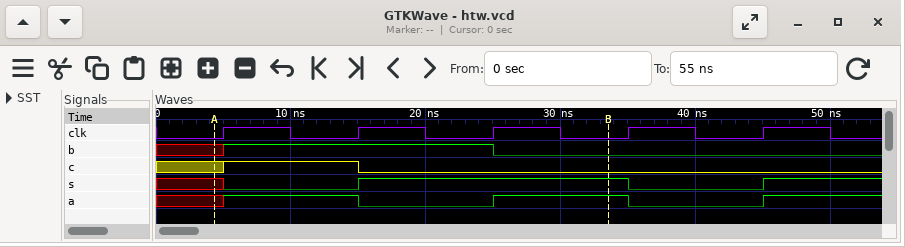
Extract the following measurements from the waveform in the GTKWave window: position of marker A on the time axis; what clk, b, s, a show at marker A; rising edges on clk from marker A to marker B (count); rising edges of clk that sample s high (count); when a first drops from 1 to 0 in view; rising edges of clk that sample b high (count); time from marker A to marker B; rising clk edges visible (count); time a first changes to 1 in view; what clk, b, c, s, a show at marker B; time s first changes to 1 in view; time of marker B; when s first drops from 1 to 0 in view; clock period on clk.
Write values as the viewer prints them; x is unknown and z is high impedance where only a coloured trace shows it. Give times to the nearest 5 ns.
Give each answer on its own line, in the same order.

5 ns
clk=0, b=x, s=x, a=x
3
2
15 ns
2
30 ns
5
5 ns
clk=0, b=0, c=0, s=1, a=1
15 ns
35 ns
35 ns
10 ns
